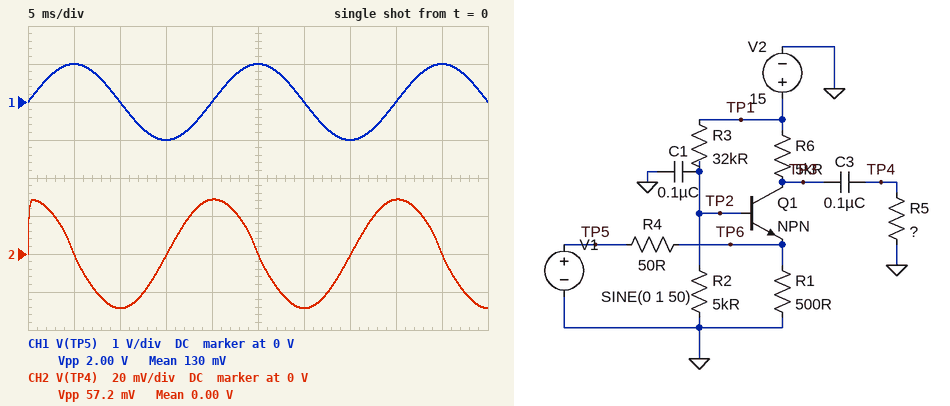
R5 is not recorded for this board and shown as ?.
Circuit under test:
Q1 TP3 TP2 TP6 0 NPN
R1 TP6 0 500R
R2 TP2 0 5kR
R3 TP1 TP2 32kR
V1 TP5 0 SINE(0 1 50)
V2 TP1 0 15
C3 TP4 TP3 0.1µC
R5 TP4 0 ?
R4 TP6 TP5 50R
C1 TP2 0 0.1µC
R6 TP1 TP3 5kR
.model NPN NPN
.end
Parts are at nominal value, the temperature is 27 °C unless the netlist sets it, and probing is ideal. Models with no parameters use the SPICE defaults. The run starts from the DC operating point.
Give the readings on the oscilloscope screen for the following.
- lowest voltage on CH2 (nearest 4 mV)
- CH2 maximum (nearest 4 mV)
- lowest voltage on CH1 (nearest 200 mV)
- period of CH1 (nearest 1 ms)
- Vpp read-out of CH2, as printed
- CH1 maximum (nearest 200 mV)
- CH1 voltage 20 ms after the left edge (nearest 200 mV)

-28 mV
28 mV
-1.0 V
20 ms
57.2 mV
1.0 V
0 V
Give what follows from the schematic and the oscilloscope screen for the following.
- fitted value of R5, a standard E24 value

1 kΩ
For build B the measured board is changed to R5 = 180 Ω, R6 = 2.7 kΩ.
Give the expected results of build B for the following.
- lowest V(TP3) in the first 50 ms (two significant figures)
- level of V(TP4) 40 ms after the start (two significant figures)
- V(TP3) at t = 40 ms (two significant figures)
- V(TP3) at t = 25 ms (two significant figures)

-550 mV
5.2 mV
350 mV
5.6 V
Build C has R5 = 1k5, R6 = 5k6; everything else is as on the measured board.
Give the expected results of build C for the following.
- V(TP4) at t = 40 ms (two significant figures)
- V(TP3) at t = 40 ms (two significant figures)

43 mV
200 mV
